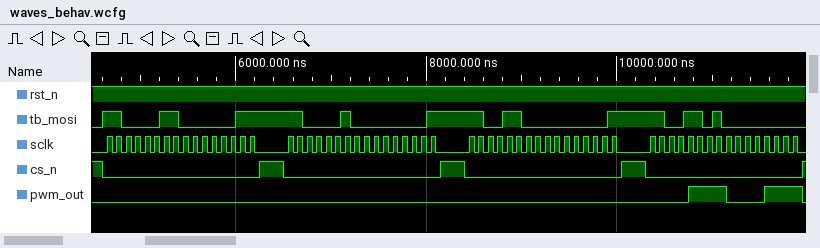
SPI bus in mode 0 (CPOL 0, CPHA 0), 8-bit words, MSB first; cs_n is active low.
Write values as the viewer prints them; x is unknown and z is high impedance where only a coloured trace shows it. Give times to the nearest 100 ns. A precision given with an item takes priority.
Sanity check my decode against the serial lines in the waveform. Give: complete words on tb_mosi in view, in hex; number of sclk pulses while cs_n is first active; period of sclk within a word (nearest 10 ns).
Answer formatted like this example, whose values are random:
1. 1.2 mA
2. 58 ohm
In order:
1. C3, 03, C2, 01, CC, 01, CD, 00
2. 16
3. 100 ns
